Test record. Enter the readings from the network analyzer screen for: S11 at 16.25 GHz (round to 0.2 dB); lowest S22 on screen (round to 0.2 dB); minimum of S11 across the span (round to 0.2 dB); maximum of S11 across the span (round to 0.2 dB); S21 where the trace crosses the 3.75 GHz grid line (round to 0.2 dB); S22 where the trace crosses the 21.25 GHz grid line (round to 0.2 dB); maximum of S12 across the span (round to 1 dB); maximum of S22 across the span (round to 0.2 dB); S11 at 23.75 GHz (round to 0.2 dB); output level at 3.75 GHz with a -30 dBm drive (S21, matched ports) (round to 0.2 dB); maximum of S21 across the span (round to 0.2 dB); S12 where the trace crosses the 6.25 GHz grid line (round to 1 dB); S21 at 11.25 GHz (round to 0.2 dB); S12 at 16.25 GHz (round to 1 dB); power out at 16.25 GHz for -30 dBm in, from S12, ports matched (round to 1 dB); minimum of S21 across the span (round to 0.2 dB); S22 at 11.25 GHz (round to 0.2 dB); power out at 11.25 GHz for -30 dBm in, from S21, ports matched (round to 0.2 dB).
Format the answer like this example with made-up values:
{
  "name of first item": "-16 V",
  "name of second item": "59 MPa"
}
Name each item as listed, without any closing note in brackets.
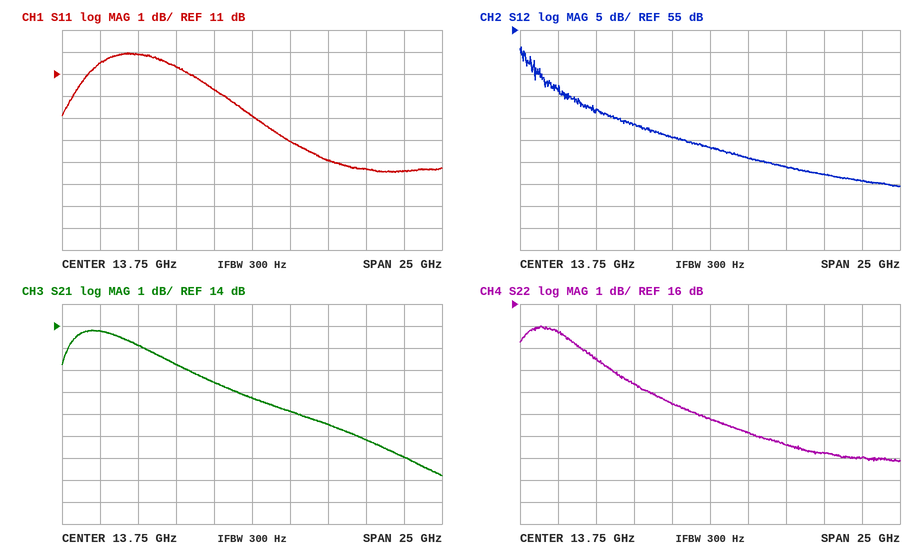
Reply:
{
  "S11 at 16.25 GHz": "8.0 dB",
  "lowest S22 on screen": "8.8 dB",
  "minimum of S11 across the span": "6.6 dB",
  "maximum of S11 across the span": "12.0 dB",
  "S21 where the trace crosses the 3.75 GHz grid line": "13.8 dB",
  "S22 where the trace crosses the 21.25 GHz grid line": "9.2 dB",
  "maximum of S12 across the span": "51 dB",
  "maximum of S22 across the span": "15.0 dB",
  "S11 at 23.75 GHz": "6.6 dB",
  "output level at 3.75 GHz with a -30 dBm drive (S21, matched ports)": "-16.2 dBm",
  "maximum of S21 across the span": "13.8 dB",
  "S12 where the trace crosses the 6.25 GHz grid line": "37 dB",
  "S21 at 11.25 GHz": "11.4 dB",
  "S12 at 16.25 GHz": "26 dB",
  "power out at 16.25 GHz for -30 dBm in, from S12, ports matched": "-4 dBm",
  "minimum of S21 across the span": "7.2 dB",
  "S22 at 11.25 GHz": "11.4 dB",
  "power out at 11.25 GHz for -30 dBm in, from S21, ports matched": "-18.6 dBm"
}
